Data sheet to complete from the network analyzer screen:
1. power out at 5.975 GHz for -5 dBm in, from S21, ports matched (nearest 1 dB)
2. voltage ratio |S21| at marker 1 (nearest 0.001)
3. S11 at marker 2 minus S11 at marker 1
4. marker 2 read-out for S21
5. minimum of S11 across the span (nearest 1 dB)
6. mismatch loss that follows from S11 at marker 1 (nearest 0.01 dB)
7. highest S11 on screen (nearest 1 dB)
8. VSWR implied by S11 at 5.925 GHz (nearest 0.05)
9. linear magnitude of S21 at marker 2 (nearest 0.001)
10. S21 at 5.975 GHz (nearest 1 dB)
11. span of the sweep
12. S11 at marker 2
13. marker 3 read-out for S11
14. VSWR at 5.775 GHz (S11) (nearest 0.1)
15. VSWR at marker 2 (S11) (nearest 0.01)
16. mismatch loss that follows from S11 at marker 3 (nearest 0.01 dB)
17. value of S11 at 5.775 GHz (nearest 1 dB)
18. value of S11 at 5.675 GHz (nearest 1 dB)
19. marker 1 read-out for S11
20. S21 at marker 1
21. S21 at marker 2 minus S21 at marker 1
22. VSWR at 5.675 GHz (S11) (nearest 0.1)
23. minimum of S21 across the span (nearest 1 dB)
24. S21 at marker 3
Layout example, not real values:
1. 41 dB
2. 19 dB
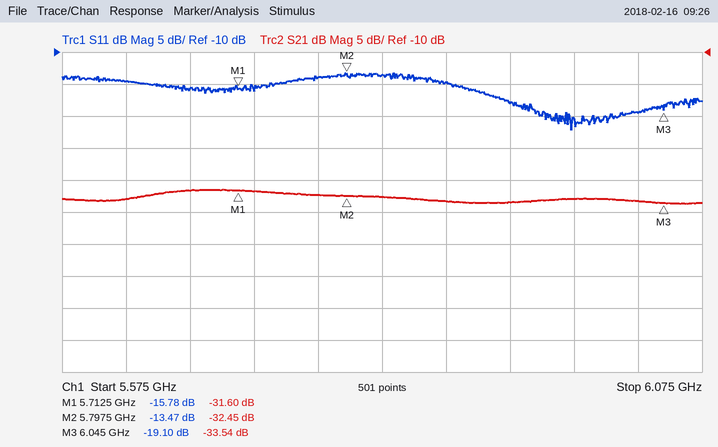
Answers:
1. -38 dBm
2. 0.026
3. 2.31 dB
4. -32.45 dB
5. -22 dB
6. 0.12 dB
7. -13 dB
8. 1.30
9. 0.024
10. -33 dB
11. 500 MHz
12. -13.47 dB
13. -19.10 dB
14. 1.5
15. 1.54
16. 0.05 dB
17. -14 dB
18. -16 dB
19. -15.78 dB
20. -31.60 dB
21. -0.85 dB
22. 1.4
23. -34 dB
24. -33.54 dB
